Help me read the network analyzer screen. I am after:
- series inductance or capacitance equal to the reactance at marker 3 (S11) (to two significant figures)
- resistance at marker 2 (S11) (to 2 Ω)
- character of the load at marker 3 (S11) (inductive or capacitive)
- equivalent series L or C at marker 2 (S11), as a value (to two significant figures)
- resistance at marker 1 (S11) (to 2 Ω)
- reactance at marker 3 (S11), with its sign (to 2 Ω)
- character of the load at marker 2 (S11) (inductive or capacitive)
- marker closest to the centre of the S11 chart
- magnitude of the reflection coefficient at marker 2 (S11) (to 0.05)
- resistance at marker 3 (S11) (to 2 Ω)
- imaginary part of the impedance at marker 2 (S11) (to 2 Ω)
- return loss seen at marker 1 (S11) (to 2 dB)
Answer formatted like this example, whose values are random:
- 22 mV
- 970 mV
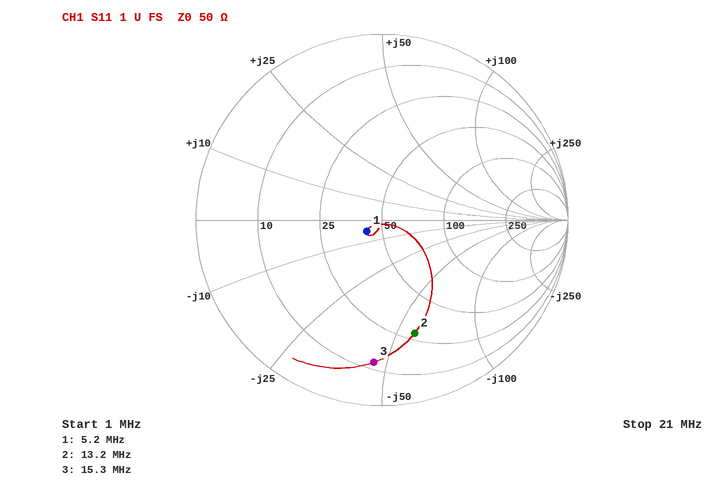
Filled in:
- 230 pF
- 28 Ω
- capacitive
- 210 pF
- 42 Ω
- -46 Ω
- capacitive
- marker 1
- 0.65
- 12 Ω
- -58 Ω
- 20 dB
